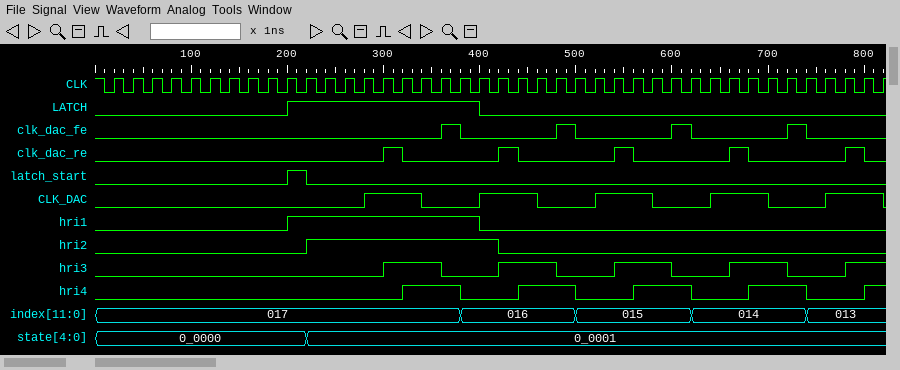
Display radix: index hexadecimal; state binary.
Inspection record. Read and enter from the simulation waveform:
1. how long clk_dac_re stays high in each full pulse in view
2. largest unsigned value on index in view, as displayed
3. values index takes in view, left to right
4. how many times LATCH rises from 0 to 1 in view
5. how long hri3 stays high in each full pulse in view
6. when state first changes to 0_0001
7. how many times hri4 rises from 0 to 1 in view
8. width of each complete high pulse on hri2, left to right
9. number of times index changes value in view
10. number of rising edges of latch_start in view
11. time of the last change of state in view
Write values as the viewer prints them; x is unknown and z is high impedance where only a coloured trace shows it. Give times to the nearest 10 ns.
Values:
20 ns, 20 ns, 20 ns, 20 ns, 20 ns
017
017, 016, 015, 014, 013
1
60 ns, 60 ns, 60 ns, 60 ns
220 ns
5
200 ns
4
1
220 ns
